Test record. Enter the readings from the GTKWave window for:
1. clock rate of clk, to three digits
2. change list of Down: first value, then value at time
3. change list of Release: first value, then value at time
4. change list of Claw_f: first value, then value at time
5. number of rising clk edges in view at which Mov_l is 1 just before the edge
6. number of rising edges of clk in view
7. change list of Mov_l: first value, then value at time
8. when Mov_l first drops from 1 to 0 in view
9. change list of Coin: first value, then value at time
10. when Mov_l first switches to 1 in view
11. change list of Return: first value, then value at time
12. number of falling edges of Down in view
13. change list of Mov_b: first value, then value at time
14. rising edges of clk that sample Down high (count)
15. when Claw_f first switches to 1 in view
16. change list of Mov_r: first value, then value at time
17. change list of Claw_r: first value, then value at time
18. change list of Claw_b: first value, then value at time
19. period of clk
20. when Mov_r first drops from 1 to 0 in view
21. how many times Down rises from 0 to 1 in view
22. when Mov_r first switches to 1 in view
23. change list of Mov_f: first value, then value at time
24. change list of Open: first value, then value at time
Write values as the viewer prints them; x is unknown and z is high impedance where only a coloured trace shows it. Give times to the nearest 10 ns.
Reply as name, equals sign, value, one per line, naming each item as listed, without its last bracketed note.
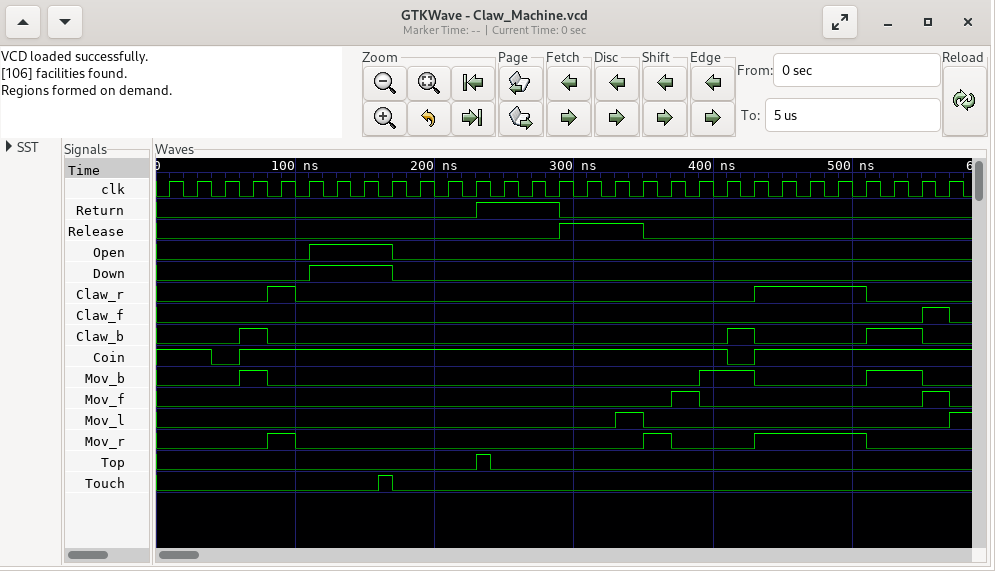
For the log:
clock rate of clk, to three digits = 50.0 MHz
change list of Down: first value, then value at time = 0, 1 at 110 ns, 0 at 170 ns
change list of Release: first value, then value at time = 0, 1 at 290 ns, 0 at 350 ns
change list of Claw_f: first value, then value at time = 0, 1 at 550 ns, 0 at 570 ns
number of rising clk edges in view at which Mov_l is 1 just before the edge = 1
number of rising edges of clk in view = 29
change list of Mov_l: first value, then value at time = 0, 1 at 330 ns, 0 at 350 ns, 1 at 570 ns
when Mov_l first drops from 1 to 0 in view = 350 ns
change list of Coin: first value, then value at time = 1, 0 at 40 ns, 1 at 60 ns, 0 at 410 ns, 1 at 430 ns
when Mov_l first switches to 1 in view = 330 ns
change list of Return: first value, then value at time = 0, 1 at 230 ns, 0 at 290 ns
number of falling edges of Down in view = 1
change list of Mov_b: first value, then value at time = 0, 1 at 60 ns, 0 at 80 ns, 1 at 390 ns, 0 at 430 ns, 1 at 510 ns, 0 at 550 ns
rising edges of clk that sample Down high = 3
when Claw_f first switches to 1 in view = 550 ns
change list of Mov_r: first value, then value at time = 0, 1 at 80 ns, 0 at 100 ns, 1 at 350 ns, 0 at 370 ns, 1 at 430 ns, 0 at 510 ns
change list of Claw_r: first value, then value at time = 0, 1 at 80 ns, 0 at 100 ns, 1 at 430 ns, 0 at 510 ns
change list of Claw_b: first value, then value at time = 0, 1 at 60 ns, 0 at 80 ns, 1 at 410 ns, 0 at 430 ns, 1 at 510 ns, 0 at 550 ns
period of clk = 20 ns
when Mov_r first drops from 1 to 0 in view = 100 ns
how many times Down rises from 0 to 1 in view = 1
when Mov_r first switches to 1 in view = 80 ns
change list of Mov_f: first value, then value at time = 0, 1 at 370 ns, 0 at 390 ns, 1 at 550 ns, 0 at 570 ns
change list of Open: first value, then value at time = 0, 1 at 110 ns, 0 at 170 ns
